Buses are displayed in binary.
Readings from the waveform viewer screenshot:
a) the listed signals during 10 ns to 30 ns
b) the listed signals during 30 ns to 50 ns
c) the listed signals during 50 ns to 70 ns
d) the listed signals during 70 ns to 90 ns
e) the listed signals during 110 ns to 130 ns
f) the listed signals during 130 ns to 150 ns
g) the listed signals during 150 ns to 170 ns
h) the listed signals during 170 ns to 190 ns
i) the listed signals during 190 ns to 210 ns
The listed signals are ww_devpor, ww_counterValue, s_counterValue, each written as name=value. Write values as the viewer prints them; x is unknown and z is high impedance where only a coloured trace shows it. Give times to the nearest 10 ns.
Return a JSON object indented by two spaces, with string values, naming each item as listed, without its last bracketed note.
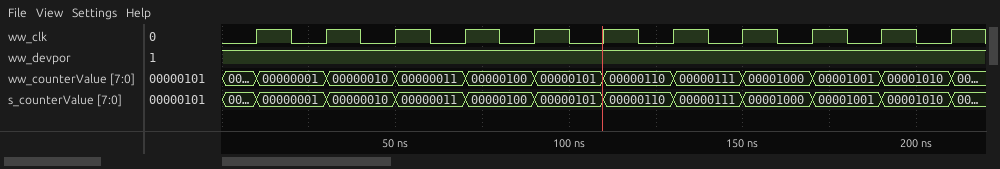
{
  "the listed signals during 10 ns to 30 ns": "ww_devpor=1, ww_counterValue=00000001, s_counterValue=00000001",
  "the listed signals during 30 ns to 50 ns": "ww_devpor=1, ww_counterValue=00000010, s_counterValue=00000010",
  "the listed signals during 50 ns to 70 ns": "ww_devpor=1, ww_counterValue=00000011, s_counterValue=00000011",
  "the listed signals during 70 ns to 90 ns": "ww_devpor=1, ww_counterValue=00000100, s_counterValue=00000100",
  "the listed signals during 110 ns to 130 ns": "ww_devpor=1, ww_counterValue=00000110, s_counterValue=00000110",
  "the listed signals during 130 ns to 150 ns": "ww_devpor=1, ww_counterValue=00000111, s_counterValue=00000111",
  "the listed signals during 150 ns to 170 ns": "ww_devpor=1, ww_counterValue=00001000, s_counterValue=00001000",
  "the listed signals during 170 ns to 190 ns": "ww_devpor=1, ww_counterValue=00001001, s_counterValue=00001001",
  "the listed signals during 190 ns to 210 ns": "ww_devpor=1, ww_counterValue=00001010, s_counterValue=00001010"
}
